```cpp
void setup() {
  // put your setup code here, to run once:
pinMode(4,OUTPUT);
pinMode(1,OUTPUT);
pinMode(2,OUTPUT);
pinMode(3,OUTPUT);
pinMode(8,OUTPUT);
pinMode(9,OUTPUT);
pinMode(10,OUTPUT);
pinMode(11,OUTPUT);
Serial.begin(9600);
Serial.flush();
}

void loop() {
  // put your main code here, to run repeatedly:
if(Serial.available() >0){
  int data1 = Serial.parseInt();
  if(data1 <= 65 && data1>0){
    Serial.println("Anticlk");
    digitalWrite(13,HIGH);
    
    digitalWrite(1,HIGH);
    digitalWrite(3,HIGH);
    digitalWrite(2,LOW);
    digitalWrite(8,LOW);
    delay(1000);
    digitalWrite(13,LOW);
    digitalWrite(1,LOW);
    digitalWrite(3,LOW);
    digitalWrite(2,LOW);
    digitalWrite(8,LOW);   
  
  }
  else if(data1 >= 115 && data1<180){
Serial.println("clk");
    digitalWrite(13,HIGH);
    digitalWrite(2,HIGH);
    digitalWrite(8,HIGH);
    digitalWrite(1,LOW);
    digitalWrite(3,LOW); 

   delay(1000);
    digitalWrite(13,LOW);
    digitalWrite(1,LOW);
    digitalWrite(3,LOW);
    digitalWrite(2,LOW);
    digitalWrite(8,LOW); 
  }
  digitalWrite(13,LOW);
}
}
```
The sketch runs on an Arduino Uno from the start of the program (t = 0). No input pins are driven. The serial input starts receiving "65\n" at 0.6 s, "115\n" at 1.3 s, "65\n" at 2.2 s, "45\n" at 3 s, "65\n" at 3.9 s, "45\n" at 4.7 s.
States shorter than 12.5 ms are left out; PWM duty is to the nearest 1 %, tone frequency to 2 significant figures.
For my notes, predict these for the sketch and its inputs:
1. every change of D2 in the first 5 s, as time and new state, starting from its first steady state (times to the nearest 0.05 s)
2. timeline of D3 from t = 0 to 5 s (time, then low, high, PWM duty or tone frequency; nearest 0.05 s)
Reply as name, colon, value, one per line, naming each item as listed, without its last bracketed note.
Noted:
every change of D2 in the first 5 s, as time and new state, starting from its first steady state: 0 s low; 1.6 s high; 2.6 s low
timeline of D3 from t = 0 to 5 s: 0 s low; 0.6 s high; 1.6 s low; 2.6 s high
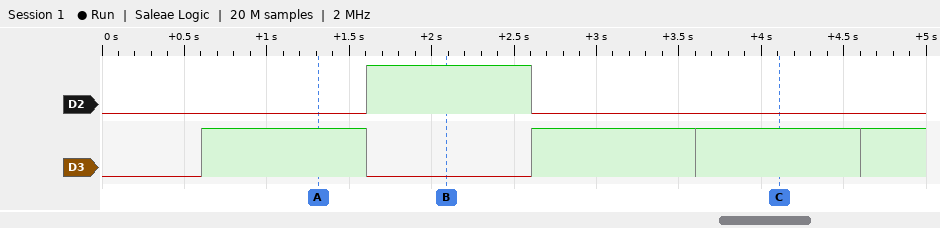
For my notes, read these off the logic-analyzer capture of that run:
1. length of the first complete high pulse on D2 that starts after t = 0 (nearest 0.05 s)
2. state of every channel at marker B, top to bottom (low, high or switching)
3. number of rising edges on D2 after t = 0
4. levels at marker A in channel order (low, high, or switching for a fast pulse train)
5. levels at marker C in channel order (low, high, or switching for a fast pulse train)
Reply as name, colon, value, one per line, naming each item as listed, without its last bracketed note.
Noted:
length of the first complete high pulse on D2 that starts after t = 0: 1.00 s
state of every channel at marker B, top to bottom: D2 high, D3 low
number of rising edges on D2 after t = 0: 1
levels at marker A in channel order: D2 low, D3 high
levels at marker C in channel order: D2 low, D3 high
